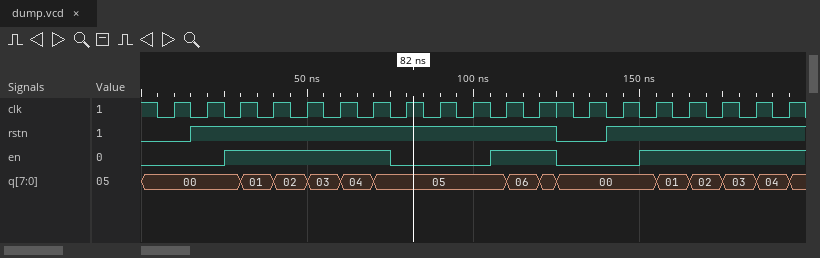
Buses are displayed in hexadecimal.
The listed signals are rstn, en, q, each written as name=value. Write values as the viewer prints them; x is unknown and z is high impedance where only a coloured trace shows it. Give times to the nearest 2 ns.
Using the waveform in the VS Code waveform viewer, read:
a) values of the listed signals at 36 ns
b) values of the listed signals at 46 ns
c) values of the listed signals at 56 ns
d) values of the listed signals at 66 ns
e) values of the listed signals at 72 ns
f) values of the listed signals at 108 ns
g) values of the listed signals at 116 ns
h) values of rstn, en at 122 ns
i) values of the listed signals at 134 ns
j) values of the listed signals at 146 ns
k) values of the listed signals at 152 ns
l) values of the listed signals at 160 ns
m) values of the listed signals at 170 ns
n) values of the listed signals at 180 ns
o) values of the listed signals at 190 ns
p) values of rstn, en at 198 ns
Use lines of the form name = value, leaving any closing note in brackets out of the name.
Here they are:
values of the listed signals at 36 ns = rstn=1, en=1, q=01
values of the listed signals at 46 ns = rstn=1, en=1, q=02
values of the listed signals at 56 ns = rstn=1, en=1, q=03
values of the listed signals at 66 ns = rstn=1, en=1, q=04
values of the listed signals at 72 ns = rstn=1, en=1, q=05
values of the listed signals at 108 ns = rstn=1, en=1, q=05
values of the listed signals at 116 ns = rstn=1, en=1, q=06
values of rstn, en at 122 ns = rstn=1, en=1
values of the listed signals at 134 ns = rstn=0, en=0, q=00
values of the listed signals at 146 ns = rstn=1, en=0, q=00
values of the listed signals at 152 ns = rstn=1, en=1, q=00
values of the listed signals at 160 ns = rstn=1, en=1, q=01
values of the listed signals at 170 ns = rstn=1, en=1, q=02
values of the listed signals at 180 ns = rstn=1, en=1, q=03
values of the listed signals at 190 ns = rstn=1, en=1, q=04
values of rstn, en at 198 ns = rstn=1, en=1
